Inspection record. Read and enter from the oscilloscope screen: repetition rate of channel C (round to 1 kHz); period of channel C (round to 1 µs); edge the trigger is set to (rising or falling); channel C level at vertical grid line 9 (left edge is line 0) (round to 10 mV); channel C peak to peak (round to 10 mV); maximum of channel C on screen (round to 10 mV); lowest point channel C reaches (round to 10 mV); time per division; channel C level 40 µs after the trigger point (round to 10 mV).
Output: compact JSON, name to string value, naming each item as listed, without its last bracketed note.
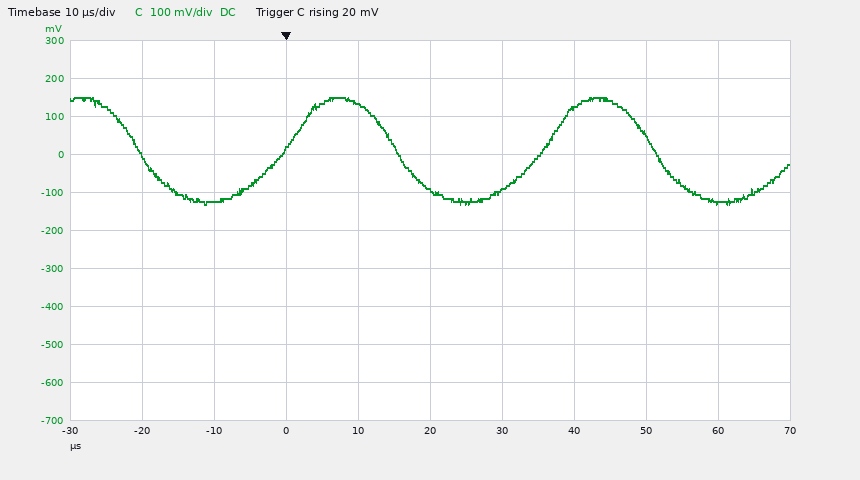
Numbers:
{"repetition rate of channel C": "28 kHz", "period of channel C": "36 µs", "edge the trigger is set to": "rising", "channel C level at vertical grid line 9 (left edge is line 0)": "-130 mV", "channel C peak to peak": "280 mV", "maximum of channel C on screen": "150 mV", "lowest point channel C reaches": "-130 mV", "time per division": "10 µs", "channel C level 40 µs after the trigger point": "120 mV"}
